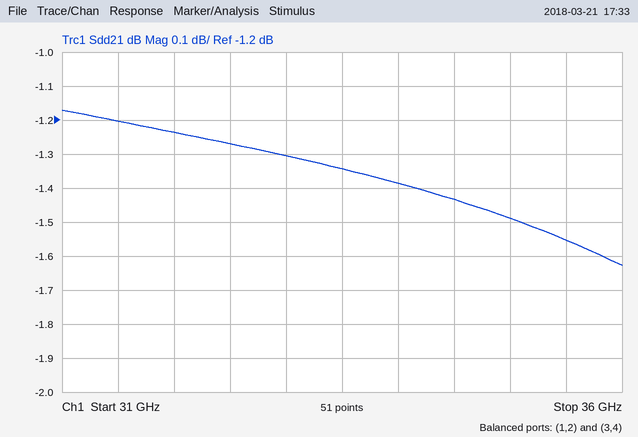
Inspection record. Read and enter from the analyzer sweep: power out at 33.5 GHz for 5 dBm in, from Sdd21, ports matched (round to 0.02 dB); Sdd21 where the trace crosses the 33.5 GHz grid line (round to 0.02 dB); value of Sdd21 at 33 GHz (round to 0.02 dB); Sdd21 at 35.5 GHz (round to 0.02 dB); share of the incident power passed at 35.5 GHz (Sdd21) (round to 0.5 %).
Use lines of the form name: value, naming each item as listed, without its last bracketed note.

power out at 33.5 GHz for 5 dBm in, from Sdd21, ports matched: 3.66 dBm
Sdd21 where the trace crosses the 33.5 GHz grid line: -1.34 dB
value of Sdd21 at 33 GHz: -1.30 dB
Sdd21 at 35.5 GHz: -1.56 dB
share of the incident power passed at 35.5 GHz (Sdd21): 70.0 %
